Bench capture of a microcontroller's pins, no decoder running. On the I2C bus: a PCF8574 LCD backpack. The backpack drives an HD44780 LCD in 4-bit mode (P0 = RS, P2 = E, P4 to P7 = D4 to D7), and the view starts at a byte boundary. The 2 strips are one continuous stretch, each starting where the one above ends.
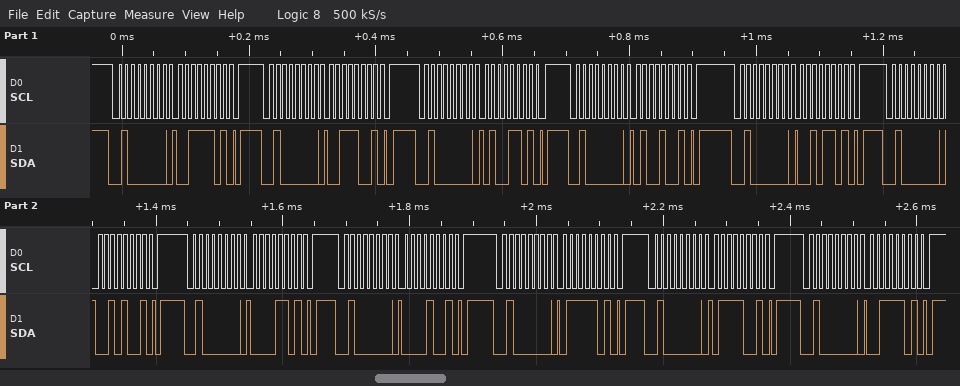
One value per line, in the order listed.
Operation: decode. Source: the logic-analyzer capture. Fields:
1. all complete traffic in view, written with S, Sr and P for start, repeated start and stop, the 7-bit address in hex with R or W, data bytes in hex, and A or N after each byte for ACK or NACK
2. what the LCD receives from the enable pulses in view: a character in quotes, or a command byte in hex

S 20W A 3D A P S 20W A 39 A P S 20W A 4D A P S 20W A 49 A P S 20W A 2D A P S 20W A 29 A P S 20W A 0D A P S 20W A 09 A P S 20W A 7D A P S 20W A 79 A P S 20W A 3D A P
'4' ' '
